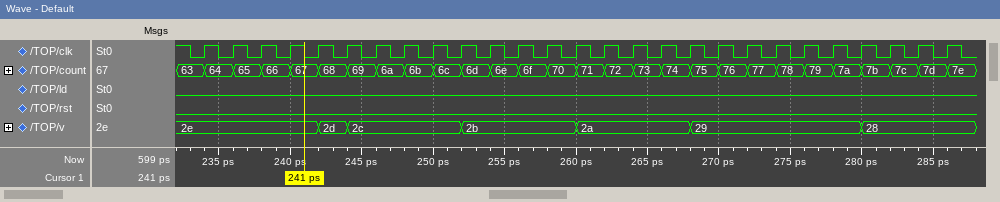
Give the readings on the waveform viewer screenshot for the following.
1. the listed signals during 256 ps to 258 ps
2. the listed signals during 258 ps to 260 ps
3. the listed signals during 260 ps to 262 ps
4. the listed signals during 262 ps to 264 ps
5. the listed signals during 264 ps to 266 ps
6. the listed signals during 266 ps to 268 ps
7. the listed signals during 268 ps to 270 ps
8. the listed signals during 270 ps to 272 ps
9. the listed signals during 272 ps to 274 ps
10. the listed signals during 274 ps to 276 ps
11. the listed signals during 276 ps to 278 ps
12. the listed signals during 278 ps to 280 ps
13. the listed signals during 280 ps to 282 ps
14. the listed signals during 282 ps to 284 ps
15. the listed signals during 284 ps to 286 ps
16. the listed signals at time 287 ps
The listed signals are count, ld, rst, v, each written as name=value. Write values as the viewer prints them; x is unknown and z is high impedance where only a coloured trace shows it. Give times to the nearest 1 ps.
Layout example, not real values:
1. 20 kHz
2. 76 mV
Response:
1. count=6f, ld=0, rst=0, v=2b
2. count=70, ld=0, rst=0, v=2b
3. count=71, ld=0, rst=0, v=2a
4. count=72, ld=0, rst=0, v=2a
5. count=73, ld=0, rst=0, v=2a
6. count=74, ld=0, rst=0, v=2a
7. count=75, ld=0, rst=0, v=29
8. count=76, ld=0, rst=0, v=29
9. count=77, ld=0, rst=0, v=29
10. count=78, ld=0, rst=0, v=29
11. count=79, ld=0, rst=0, v=29
12. count=7a, ld=0, rst=0, v=29
13. count=7b, ld=0, rst=0, v=28
14. count=7c, ld=0, rst=0, v=28
15. count=7d, ld=0, rst=0, v=28
16. count=7e, ld=0, rst=0, v=28
